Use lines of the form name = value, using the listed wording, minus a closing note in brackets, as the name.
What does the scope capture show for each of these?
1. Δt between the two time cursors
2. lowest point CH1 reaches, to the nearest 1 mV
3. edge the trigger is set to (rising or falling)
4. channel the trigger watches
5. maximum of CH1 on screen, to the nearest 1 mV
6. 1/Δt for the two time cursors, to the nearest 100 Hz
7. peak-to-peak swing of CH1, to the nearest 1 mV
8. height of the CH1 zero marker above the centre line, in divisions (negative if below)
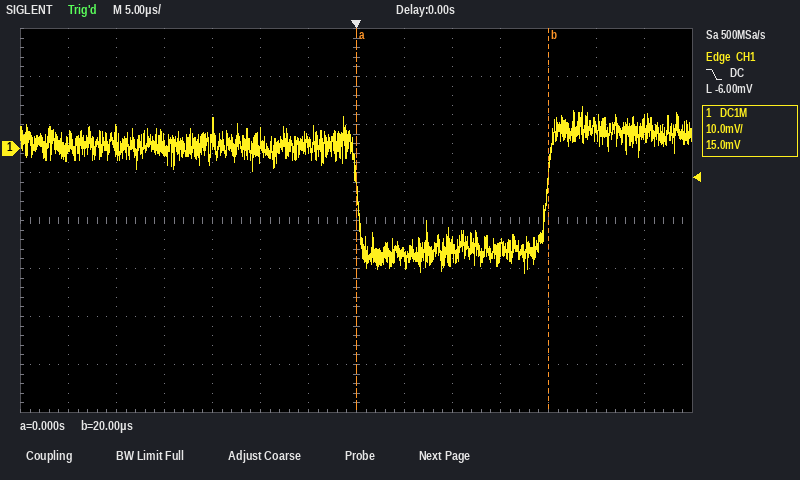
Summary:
Δt between the two time cursors = 20.0 µs
lowest point CH1 reaches, to the nearest 1 mV = -26 mV
edge the trigger is set to = falling
channel the trigger watches = CH1
maximum of CH1 on screen, to the nearest 1 mV = 9 mV
1/Δt for the two time cursors, to the nearest 100 Hz = 50.0 kHz
peak-to-peak swing of CH1, to the nearest 1 mV = 35 mV
height of the CH1 zero marker above the centre line, in divisions = +1.5 div
